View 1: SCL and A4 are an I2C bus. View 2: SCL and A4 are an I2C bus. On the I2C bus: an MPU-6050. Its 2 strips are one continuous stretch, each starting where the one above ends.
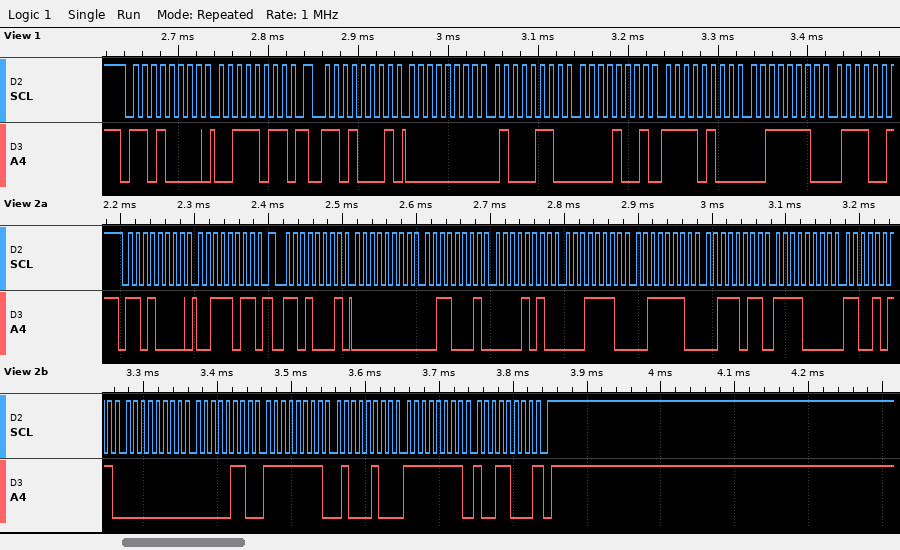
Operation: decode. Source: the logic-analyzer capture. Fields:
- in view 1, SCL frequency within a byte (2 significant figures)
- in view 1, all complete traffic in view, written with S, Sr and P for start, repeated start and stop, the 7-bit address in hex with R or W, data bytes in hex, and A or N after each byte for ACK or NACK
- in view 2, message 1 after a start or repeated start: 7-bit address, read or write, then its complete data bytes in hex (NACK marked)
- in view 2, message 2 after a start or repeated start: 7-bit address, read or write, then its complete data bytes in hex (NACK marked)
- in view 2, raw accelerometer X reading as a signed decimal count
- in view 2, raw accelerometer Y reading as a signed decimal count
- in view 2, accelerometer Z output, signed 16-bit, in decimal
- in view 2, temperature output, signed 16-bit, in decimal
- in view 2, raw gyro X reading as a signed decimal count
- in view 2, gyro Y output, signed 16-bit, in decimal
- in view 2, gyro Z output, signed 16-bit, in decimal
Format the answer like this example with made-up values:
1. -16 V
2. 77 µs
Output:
1. 100 kHz
2. S 68W A 3B A Sr 68R A 00 A 46 A 09 A F4 A 3E A
3. 0x68 write: 3B
4. 0x68 read: 00 31 0A 1E 3E 3B F0 CB 00 06 FF 44 FF 98 NACK
5. 49
6. 2590
7. 15931
8. -3893
9. 6
10. -188
11. -104
